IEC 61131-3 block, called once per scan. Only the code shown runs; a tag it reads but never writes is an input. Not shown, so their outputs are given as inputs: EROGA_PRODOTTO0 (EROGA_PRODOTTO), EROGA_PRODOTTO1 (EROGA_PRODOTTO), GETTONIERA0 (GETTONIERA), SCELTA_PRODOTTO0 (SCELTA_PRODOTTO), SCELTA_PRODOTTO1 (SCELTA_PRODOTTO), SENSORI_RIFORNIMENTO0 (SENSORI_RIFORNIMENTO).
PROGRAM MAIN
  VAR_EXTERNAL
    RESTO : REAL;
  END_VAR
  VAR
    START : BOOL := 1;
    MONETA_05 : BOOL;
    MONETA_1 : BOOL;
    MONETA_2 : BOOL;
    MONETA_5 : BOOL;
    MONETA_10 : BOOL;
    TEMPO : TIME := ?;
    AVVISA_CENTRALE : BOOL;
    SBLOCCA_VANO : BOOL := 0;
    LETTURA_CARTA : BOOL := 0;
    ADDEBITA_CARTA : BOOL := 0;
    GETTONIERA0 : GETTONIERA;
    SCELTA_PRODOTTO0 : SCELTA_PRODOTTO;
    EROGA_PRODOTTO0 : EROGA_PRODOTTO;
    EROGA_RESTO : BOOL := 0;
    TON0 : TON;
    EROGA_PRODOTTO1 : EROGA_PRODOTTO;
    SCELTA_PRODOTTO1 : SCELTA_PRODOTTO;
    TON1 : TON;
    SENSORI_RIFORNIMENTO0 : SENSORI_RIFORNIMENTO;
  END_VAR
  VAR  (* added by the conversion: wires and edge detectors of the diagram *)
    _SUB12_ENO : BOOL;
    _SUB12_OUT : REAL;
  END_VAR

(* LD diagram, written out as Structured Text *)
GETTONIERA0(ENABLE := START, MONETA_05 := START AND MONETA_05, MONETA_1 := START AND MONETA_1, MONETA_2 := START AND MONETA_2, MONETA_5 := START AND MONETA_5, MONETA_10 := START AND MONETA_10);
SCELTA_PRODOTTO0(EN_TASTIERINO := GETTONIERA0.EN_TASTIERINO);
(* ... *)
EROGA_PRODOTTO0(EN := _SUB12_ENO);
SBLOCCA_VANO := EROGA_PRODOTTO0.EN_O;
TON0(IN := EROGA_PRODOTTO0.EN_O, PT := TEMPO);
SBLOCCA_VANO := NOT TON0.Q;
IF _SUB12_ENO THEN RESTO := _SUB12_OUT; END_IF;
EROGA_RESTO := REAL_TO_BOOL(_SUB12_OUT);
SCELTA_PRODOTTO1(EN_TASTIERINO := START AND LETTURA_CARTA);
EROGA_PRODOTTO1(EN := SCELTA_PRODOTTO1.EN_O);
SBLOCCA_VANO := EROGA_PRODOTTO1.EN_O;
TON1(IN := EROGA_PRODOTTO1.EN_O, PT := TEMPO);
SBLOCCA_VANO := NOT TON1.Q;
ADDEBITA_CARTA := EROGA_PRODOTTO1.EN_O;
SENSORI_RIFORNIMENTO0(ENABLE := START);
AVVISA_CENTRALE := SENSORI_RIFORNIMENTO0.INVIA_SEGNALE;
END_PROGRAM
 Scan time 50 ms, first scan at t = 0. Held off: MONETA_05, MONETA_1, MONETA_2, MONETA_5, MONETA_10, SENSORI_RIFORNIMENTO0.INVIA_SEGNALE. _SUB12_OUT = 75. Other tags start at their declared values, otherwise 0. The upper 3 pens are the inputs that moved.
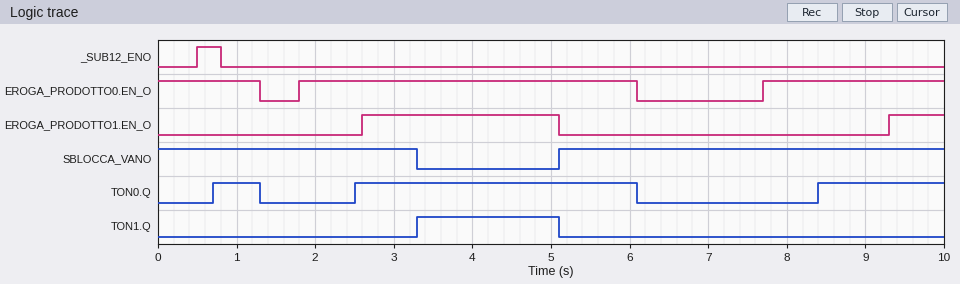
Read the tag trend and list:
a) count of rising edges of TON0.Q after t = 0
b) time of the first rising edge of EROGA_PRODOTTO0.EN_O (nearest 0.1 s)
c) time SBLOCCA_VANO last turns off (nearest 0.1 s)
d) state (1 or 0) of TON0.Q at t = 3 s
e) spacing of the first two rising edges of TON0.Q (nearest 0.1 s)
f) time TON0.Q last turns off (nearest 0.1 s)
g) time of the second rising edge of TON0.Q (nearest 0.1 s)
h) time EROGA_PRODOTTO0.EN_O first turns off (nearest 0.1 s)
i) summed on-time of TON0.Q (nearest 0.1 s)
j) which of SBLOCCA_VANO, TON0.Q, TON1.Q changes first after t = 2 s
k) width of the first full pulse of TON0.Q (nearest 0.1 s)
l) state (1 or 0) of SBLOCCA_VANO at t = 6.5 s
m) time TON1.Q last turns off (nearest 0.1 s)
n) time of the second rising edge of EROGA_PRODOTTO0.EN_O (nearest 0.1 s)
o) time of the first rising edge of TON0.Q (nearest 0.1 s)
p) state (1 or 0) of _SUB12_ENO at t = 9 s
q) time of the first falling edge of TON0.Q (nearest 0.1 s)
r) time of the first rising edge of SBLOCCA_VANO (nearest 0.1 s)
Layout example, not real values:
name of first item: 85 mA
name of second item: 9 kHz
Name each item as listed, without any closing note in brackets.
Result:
count of rising edges of TON0.Q after t = 0: 3
time of the first rising edge of EROGA_PRODOTTO0.EN_O: 1.8 s
time SBLOCCA_VANO last turns off: 3.3 s
state (1 or 0) of TON0.Q at t = 3 s: 1
spacing of the first two rising edges of TON0.Q: 1.8 s
time TON0.Q last turns off: 6.1 s
time of the second rising edge of TON0.Q: 2.5 s
time EROGA_PRODOTTO0.EN_O first turns off: 1.3 s
summed on-time of TON0.Q: 5.8 s
which of SBLOCCA_VANO, TON0.Q, TON1.Q changes first after t = 2 s: TON0.Q
width of the first full pulse of TON0.Q: 0.6 s
state (1 or 0) of SBLOCCA_VANO at t = 6.5 s: 1
time TON1.Q last turns off: 5.1 s
time of the second rising edge of EROGA_PRODOTTO0.EN_O: 7.7 s
time of the first rising edge of TON0.Q: 0.7 s
state (1 or 0) of _SUB12_ENO at t = 9 s: 0
time of the first falling edge of TON0.Q: 1.3 s
time of the first rising edge of SBLOCCA_VANO: 5.1 s
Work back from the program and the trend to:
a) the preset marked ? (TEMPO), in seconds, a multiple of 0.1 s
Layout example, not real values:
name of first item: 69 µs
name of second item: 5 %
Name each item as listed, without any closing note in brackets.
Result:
the preset marked ? (TEMPO), in seconds, a multiple of 0.1 s: 0.7 s
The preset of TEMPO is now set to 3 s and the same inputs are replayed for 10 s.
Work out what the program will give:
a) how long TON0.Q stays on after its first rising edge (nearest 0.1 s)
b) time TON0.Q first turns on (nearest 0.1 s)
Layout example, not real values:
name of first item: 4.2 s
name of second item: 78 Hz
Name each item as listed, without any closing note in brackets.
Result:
how long TON0.Q stays on after its first rising edge: 1.3 s
time TON0.Q first turns on: 4.8 s
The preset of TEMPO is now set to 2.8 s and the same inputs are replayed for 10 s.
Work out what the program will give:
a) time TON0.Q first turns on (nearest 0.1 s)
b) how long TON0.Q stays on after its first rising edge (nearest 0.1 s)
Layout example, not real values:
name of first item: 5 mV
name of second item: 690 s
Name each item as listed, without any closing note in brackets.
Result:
time TON0.Q first turns on: 4.6 s
how long TON0.Q stays on after its first rising edge: 1.5 s
